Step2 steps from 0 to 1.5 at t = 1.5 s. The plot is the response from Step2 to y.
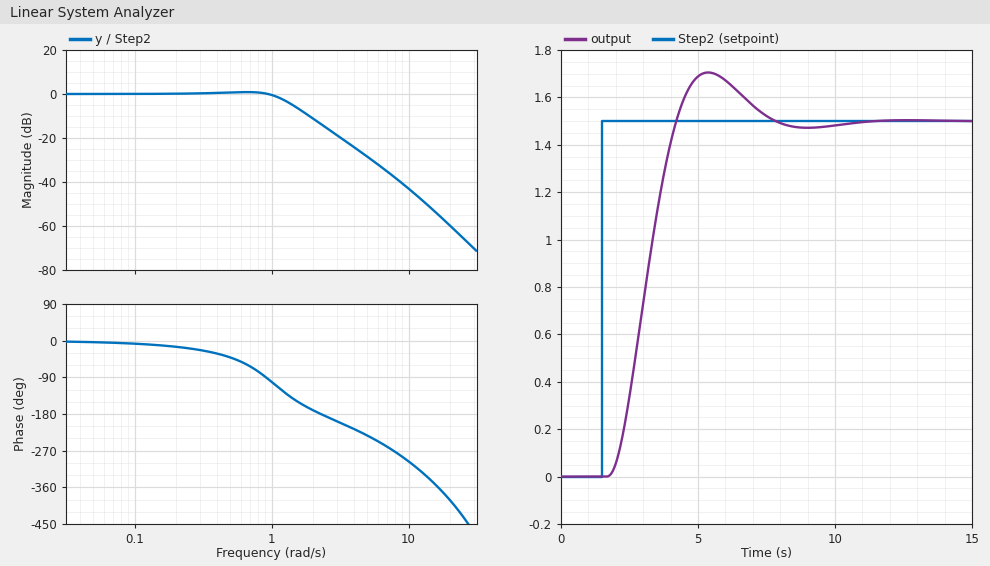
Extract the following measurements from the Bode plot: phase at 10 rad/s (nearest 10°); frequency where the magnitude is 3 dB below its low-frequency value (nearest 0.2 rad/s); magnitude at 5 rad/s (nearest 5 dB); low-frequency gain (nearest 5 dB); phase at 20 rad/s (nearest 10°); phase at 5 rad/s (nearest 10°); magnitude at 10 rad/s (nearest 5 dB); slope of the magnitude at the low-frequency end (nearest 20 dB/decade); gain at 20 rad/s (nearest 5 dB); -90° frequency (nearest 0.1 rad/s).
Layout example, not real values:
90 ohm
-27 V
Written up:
-300°
1.2 rad/s
-30 dB
0 dB
-390°
-230°
-45 dB
0 dB/decade
-60 dB
0.9 rad/s
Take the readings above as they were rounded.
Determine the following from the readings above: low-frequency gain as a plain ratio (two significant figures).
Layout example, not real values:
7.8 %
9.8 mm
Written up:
1.0
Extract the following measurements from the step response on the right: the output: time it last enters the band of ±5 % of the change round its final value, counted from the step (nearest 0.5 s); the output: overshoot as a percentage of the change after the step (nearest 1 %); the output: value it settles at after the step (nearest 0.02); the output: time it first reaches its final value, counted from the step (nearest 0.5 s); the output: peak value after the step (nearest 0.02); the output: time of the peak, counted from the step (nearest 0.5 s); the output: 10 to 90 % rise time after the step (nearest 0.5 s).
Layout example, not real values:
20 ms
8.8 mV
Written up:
5.5 s
14 %
1.50
2.5 s
1.70
4.0 s
1.5 s
